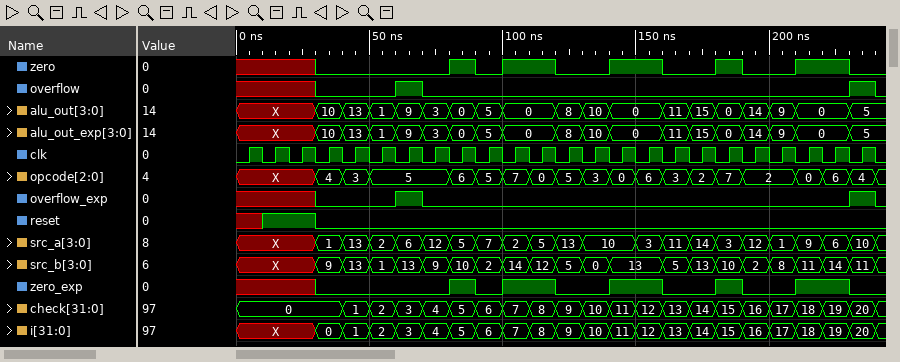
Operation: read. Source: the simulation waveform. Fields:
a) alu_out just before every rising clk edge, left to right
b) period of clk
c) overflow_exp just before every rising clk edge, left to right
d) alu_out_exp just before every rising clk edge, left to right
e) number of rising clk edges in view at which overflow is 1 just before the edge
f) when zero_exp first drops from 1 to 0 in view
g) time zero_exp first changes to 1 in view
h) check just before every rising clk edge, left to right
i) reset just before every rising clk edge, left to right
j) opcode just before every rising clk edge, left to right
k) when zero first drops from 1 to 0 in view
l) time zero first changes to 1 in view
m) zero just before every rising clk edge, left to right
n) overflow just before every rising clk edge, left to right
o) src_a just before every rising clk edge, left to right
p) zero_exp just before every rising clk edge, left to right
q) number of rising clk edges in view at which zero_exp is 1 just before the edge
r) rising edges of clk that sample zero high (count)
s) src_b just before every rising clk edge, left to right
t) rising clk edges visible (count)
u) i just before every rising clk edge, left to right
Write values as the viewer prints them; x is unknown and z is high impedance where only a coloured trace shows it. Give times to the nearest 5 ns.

X, X, X, 10, 13, 1, 9, 3, 0, 5, 0, 0, 8, 10, 0, 0, 11, 15, 0, 14, 9, 0, 0, 5
10 ns
x x x 0 0 0 1 0 0 0 0 0 0 0 0 0 0 0 0 0 0 0 0 1
X, X, X, 10, 13, 1, 9, 3, 0, 5, 0, 0, 8, 10, 0, 0, 11, 15, 0, 14, 9, 0, 0, 5
2
90 ns
80 ns
0, 0, 0, 0, 1, 2, 3, 4, 5, 6, 7, 8, 9, 10, 11, 12, 13, 14, 15, 16, 17, 18, 19, 20
x 1 1 0 0 0 0 0 0 0 0 0 0 0 0 0 0 0 0 0 0 0 0 0
X, X, X, 4, 3, 5, 5, 5, 6, 5, 7, 0, 5, 3, 0, 6, 3, 2, 7, 2, 2, 0, 6, 4
90 ns
80 ns
x x x 0 0 0 0 0 1 0 1 1 0 0 1 1 0 0 1 0 0 1 1 0
x x x 0 0 0 1 0 0 0 0 0 0 0 0 0 0 0 0 0 0 0 0 1
X, X, X, 1, 13, 2, 6, 12, 5, 7, 2, 5, 13, 10, 10, 3, 11, 14, 3, 12, 1, 9, 6, 10
x x x 0 0 0 0 0 1 0 1 1 0 0 1 1 0 0 1 0 0 1 1 0
8
8
X, X, X, 9, 13, 1, 13, 9, 10, 2, 14, 12, 5, 0, 13, 13, 5, 13, 10, 2, 8, 11, 14, 11
24
X, X, X, 0, 1, 2, 3, 4, 5, 6, 7, 8, 9, 10, 11, 12, 13, 14, 15, 16, 17, 18, 19, 20
